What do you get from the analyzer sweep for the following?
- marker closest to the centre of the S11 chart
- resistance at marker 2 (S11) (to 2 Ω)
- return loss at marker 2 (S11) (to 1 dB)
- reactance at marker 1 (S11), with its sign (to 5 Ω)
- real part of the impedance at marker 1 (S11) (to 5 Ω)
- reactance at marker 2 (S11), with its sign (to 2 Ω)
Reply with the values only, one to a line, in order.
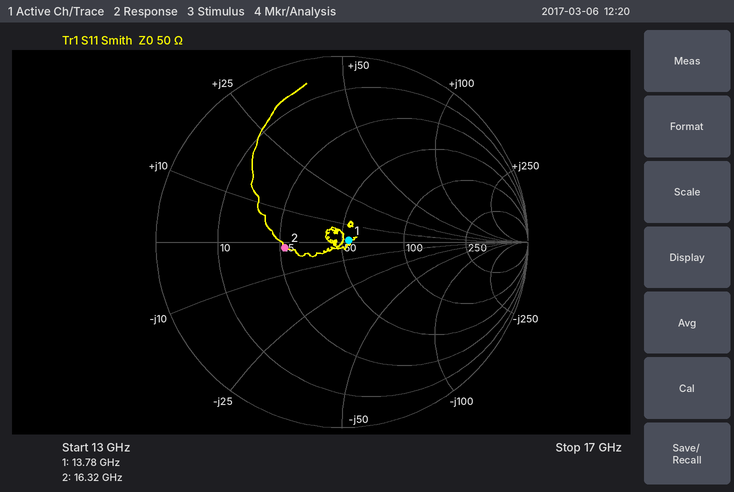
marker 1
26 Ω
10 dB
0 Ω
55 Ω
-2 Ω
